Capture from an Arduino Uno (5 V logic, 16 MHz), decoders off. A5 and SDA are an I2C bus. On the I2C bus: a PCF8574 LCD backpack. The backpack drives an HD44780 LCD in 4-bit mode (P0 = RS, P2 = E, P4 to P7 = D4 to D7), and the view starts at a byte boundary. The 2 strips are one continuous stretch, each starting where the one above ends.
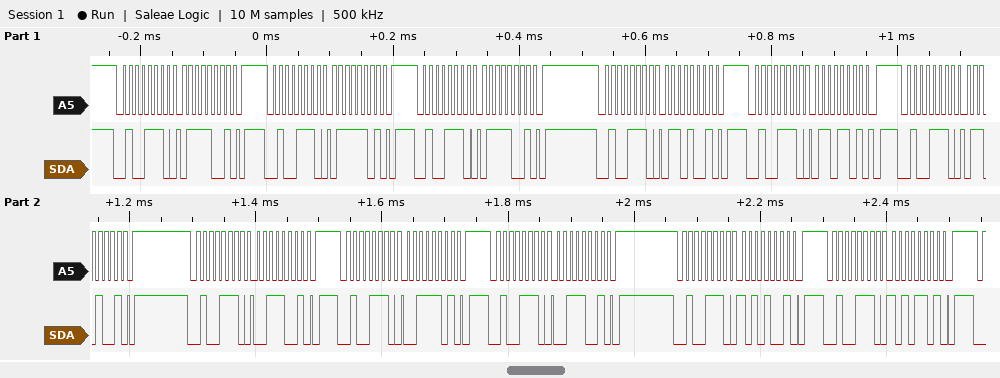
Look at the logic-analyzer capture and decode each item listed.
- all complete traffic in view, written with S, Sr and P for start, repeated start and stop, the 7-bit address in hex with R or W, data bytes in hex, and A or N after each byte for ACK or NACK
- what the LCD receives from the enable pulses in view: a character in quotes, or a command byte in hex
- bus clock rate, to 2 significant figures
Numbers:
S 27W A 79 A P S 27W A 7D A P S 27W A 79 A P S 27W A 69 A P S 27W A 6D A P S 27W A 69 A P S 27W A 39 A P S 27W A 3D A P S 27W A 39 A P S 27W A A9 A P S 27W A AD A P
'v'
100 kHz
